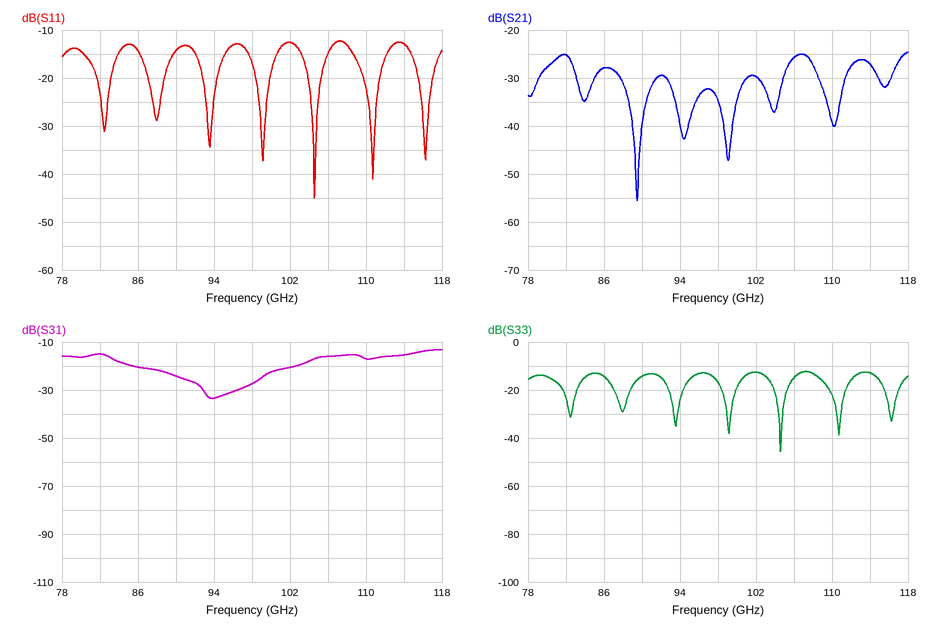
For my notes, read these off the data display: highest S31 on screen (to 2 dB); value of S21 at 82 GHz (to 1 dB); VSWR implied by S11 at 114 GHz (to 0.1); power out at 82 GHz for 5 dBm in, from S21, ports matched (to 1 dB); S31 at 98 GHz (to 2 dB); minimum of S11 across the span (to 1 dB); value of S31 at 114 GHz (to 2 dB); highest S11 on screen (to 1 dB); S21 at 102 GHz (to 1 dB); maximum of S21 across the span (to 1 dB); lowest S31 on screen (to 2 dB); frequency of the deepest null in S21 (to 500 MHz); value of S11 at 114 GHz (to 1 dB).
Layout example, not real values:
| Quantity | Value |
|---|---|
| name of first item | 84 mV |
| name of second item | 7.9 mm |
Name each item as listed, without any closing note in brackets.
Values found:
| Quantity | Value |
|---|---|
| highest S31 on screen | -14 dB |
| value of S21 at 82 GHz | -25 dB |
| VSWR implied by S11 at 114 GHz | 1.6 |
| power out at 82 GHz for 5 dBm in, from S21, ports matched | -20 dBm |
| S31 at 98 GHz | -28 dB |
| minimum of S11 across the span | -45 dB |
| value of S31 at 114 GHz | -16 dB |
| highest S11 on screen | -12 dB |
| S21 at 102 GHz | -30 dB |
| maximum of S21 across the span | -25 dB |
| lowest S31 on screen | -34 dB |
| frequency of the deepest null in S21 | 89.5 GHz |
| value of S11 at 114 GHz | -13 dB |
